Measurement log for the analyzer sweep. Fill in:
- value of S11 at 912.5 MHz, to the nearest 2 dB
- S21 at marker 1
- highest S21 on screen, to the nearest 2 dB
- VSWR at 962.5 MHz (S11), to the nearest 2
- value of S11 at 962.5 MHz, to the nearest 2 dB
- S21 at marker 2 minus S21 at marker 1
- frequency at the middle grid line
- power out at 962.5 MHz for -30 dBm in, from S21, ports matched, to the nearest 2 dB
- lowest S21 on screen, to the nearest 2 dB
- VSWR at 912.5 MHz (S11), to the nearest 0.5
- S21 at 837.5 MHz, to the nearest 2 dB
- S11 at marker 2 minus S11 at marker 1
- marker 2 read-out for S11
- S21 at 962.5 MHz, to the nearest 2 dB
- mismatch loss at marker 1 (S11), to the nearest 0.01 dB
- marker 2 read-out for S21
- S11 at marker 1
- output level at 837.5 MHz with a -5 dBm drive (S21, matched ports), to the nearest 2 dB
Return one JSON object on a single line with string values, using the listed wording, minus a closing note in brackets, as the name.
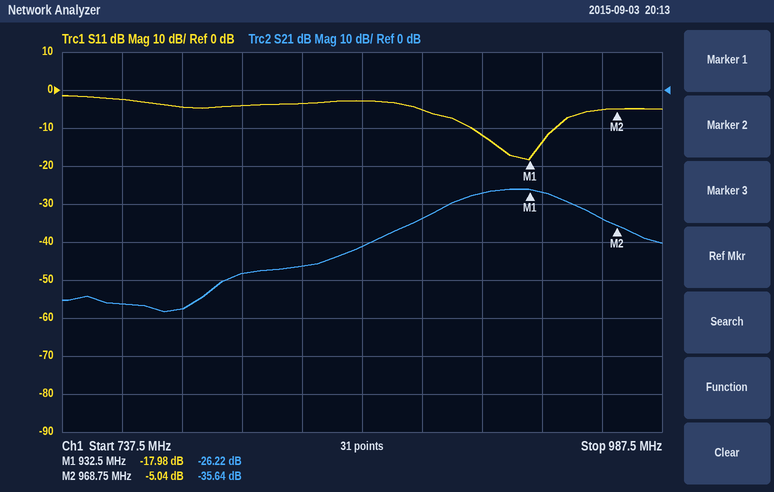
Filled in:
{"value of S11 at 912.5 MHz, to the nearest 2 dB": "-12 dB", "S21 at marker 1": "-26.22 dB", "highest S21 on screen, to the nearest 2 dB": "-26 dB", "VSWR at 962.5 MHz (S11), to the nearest 2": "4", "value of S11 at 962.5 MHz, to the nearest 2 dB": "-6 dB", "S21 at marker 2 minus S21 at marker 1": "-9.42 dB", "frequency at the middle grid line": "862.5 MHz", "power out at 962.5 MHz for -30 dBm in, from S21, ports matched, to the nearest 2 dB": "-64 dBm", "lowest S21 on screen, to the nearest 2 dB": "-58 dB", "VSWR at 912.5 MHz (S11), to the nearest 0.5": "1.5", "S21 at 837.5 MHz, to the nearest 2 dB": "-46 dB", "S11 at marker 2 minus S11 at marker 1": "12.94 dB", "marker 2 read-out for S11": "-5.04 dB", "S21 at 962.5 MHz, to the nearest 2 dB": "-34 dB", "mismatch loss at marker 1 (S11), to the nearest 0.01 dB": "0.07 dB", "marker 2 read-out for S21": "-35.64 dB", "S11 at marker 1": "-17.98 dB", "output level at 837.5 MHz with a -5 dBm drive (S21, matched ports), to the nearest 2 dB": "-52 dBm"}
